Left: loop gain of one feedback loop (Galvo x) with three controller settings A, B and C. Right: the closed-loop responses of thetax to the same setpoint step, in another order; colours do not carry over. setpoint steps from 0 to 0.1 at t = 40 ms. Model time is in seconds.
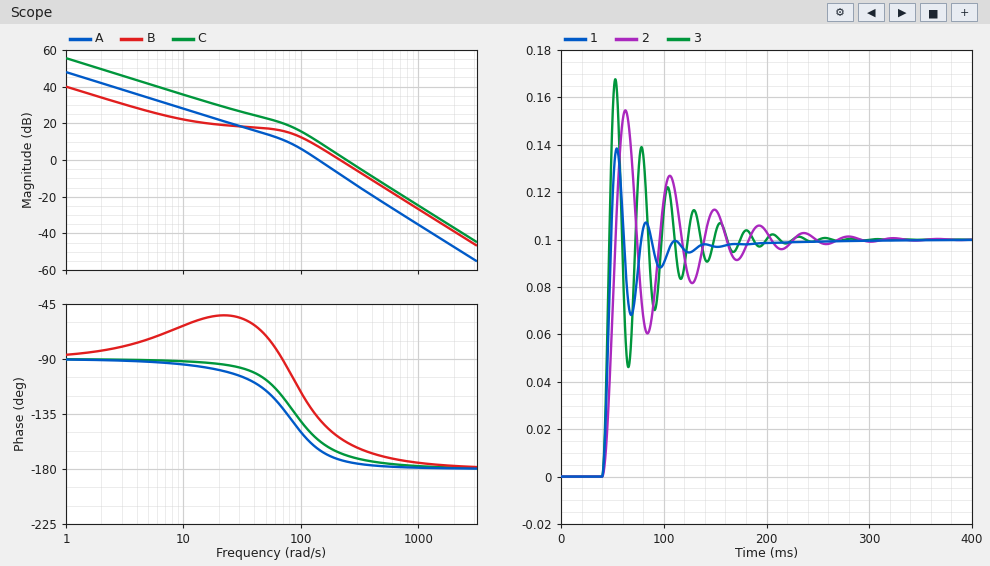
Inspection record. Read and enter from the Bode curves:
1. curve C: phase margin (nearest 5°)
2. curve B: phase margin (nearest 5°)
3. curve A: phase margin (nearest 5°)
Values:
10°
25°
15°
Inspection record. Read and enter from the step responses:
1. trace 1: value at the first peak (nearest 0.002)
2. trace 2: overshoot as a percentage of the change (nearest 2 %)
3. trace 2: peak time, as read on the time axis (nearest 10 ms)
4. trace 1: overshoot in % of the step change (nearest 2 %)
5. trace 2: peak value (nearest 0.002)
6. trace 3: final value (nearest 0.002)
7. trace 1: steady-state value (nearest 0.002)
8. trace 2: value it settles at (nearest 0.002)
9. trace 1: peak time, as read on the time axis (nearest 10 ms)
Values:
0.138
54 %
60 ms
38 %
0.154
0.100
0.100
0.100
50 ms
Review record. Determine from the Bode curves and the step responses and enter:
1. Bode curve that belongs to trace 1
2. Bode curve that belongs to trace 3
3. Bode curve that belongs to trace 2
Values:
B
C
A
